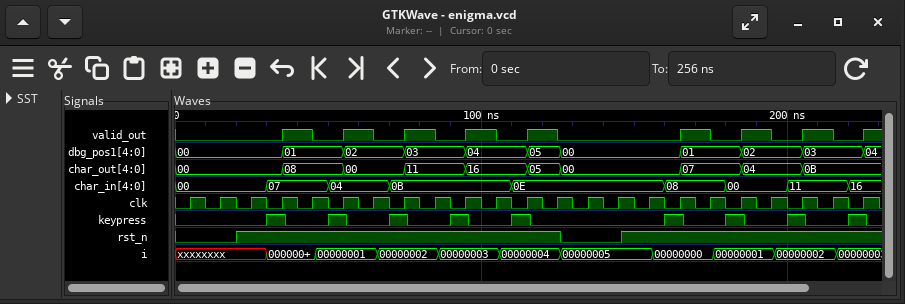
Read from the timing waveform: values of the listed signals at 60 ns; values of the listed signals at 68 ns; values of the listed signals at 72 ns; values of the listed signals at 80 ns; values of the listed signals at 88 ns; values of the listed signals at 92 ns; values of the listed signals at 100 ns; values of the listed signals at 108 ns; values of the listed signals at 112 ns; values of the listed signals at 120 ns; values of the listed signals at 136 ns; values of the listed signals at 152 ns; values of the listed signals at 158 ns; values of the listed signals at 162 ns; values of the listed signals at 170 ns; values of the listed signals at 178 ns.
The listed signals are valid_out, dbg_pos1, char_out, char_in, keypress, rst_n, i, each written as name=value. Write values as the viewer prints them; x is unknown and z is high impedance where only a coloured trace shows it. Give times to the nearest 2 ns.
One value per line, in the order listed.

valid_out=1, dbg_pos1=02, char_out=00, char_in=04, keypress=0, rst_n=1, i=00000001
valid_out=0, dbg_pos1=02, char_out=00, char_in=04, keypress=0, rst_n=1, i=00000002
valid_out=0, dbg_pos1=02, char_out=00, char_in=0B, keypress=1, rst_n=1, i=00000002
valid_out=1, dbg_pos1=03, char_out=11, char_in=0B, keypress=0, rst_n=1, i=00000002
valid_out=0, dbg_pos1=03, char_out=11, char_in=0B, keypress=0, rst_n=1, i=00000003
valid_out=0, dbg_pos1=03, char_out=11, char_in=0B, keypress=1, rst_n=1, i=00000003
valid_out=1, dbg_pos1=04, char_out=16, char_in=0B, keypress=0, rst_n=1, i=00000003
valid_out=0, dbg_pos1=04, char_out=16, char_in=0B, keypress=0, rst_n=1, i=00000004
valid_out=0, dbg_pos1=04, char_out=16, char_in=0E, keypress=1, rst_n=1, i=00000004
valid_out=1, dbg_pos1=05, char_out=05, char_in=0E, keypress=0, rst_n=1, i=00000004
valid_out=0, dbg_pos1=00, char_out=00, char_in=0E, keypress=0, rst_n=0, i=00000005
valid_out=0, dbg_pos1=00, char_out=00, char_in=0E, keypress=0, rst_n=1, i=00000005
valid_out=0, dbg_pos1=00, char_out=00, char_in=0E, keypress=0, rst_n=1, i=00000000
valid_out=0, dbg_pos1=00, char_out=00, char_in=08, keypress=1, rst_n=1, i=00000000
valid_out=1, dbg_pos1=01, char_out=07, char_in=08, keypress=0, rst_n=1, i=00000000
valid_out=0, dbg_pos1=01, char_out=07, char_in=08, keypress=0, rst_n=1, i=00000001
